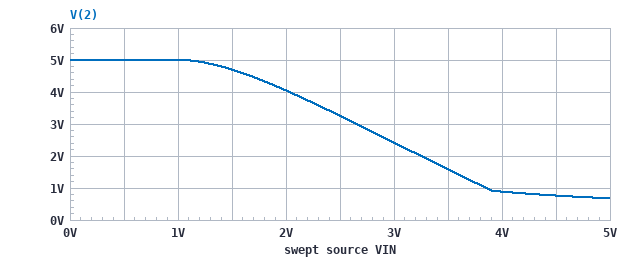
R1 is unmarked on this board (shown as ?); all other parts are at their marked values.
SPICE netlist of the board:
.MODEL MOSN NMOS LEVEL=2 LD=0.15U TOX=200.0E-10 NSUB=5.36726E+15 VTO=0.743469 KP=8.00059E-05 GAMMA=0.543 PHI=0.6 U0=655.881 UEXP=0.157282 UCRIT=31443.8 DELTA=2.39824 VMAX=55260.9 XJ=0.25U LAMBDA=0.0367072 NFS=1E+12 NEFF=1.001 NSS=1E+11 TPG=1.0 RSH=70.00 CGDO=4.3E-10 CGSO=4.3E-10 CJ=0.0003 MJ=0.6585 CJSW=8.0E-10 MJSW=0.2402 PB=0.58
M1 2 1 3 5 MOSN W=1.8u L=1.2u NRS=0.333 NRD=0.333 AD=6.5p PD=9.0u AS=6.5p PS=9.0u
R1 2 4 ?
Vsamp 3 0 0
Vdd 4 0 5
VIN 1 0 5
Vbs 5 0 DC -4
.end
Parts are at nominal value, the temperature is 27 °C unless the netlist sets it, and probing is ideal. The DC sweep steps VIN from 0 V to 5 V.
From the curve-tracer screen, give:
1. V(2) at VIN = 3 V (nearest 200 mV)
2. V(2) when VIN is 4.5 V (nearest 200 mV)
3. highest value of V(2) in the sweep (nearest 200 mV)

2.4 V
800 mV
5.0 V
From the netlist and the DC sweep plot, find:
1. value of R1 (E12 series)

18 kΩ
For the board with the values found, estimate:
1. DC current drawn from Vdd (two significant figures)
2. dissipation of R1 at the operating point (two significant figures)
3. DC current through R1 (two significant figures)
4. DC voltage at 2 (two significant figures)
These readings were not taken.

240 µA
1.0 mW
240 µA
680 mV
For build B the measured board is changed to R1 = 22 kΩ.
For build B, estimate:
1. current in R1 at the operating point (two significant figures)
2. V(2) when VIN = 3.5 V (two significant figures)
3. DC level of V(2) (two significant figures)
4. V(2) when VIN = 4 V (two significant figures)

200 µA
960 mV
560 mV
730 mV
